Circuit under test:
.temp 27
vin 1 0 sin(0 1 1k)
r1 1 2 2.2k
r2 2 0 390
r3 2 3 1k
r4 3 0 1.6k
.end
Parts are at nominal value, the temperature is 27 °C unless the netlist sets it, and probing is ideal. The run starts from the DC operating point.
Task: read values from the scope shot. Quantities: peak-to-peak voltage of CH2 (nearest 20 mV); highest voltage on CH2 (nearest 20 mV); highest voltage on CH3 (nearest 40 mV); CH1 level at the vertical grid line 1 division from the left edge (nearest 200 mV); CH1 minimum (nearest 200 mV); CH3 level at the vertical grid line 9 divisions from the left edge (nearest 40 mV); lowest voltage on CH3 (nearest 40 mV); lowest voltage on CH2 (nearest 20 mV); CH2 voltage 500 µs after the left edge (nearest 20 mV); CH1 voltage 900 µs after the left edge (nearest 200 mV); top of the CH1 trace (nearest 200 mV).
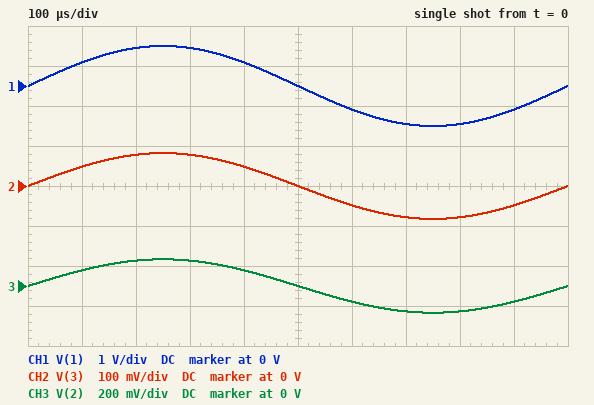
160 mV
80 mV
120 mV
600 mV
-1.0 V
-80 mV
-120 mV
-80 mV
0 V
-600 mV
1.0 V
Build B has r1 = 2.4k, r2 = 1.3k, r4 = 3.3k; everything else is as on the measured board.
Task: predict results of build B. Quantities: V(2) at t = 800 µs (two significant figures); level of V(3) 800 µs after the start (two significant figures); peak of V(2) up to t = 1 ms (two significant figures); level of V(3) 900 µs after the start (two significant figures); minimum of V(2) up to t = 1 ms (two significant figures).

-280 mV
-210 mV
290 mV
-130 mV
-290 mV
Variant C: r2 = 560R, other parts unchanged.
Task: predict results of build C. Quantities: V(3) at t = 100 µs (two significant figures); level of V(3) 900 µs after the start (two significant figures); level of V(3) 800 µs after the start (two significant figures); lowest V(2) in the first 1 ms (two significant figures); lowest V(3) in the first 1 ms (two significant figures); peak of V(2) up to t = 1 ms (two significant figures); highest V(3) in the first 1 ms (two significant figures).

63 mV
-63 mV
-100 mV
-170 mV
-110 mV
170 mV
110 mV
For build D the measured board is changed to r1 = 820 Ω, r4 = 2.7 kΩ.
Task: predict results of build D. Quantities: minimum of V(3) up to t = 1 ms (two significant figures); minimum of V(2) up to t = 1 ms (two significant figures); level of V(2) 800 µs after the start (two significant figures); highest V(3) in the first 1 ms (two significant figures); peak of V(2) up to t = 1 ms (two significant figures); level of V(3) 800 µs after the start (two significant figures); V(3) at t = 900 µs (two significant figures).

-220 mV
-300 mV
-290 mV
220 mV
300 mV
-210 mV
-130 mV
